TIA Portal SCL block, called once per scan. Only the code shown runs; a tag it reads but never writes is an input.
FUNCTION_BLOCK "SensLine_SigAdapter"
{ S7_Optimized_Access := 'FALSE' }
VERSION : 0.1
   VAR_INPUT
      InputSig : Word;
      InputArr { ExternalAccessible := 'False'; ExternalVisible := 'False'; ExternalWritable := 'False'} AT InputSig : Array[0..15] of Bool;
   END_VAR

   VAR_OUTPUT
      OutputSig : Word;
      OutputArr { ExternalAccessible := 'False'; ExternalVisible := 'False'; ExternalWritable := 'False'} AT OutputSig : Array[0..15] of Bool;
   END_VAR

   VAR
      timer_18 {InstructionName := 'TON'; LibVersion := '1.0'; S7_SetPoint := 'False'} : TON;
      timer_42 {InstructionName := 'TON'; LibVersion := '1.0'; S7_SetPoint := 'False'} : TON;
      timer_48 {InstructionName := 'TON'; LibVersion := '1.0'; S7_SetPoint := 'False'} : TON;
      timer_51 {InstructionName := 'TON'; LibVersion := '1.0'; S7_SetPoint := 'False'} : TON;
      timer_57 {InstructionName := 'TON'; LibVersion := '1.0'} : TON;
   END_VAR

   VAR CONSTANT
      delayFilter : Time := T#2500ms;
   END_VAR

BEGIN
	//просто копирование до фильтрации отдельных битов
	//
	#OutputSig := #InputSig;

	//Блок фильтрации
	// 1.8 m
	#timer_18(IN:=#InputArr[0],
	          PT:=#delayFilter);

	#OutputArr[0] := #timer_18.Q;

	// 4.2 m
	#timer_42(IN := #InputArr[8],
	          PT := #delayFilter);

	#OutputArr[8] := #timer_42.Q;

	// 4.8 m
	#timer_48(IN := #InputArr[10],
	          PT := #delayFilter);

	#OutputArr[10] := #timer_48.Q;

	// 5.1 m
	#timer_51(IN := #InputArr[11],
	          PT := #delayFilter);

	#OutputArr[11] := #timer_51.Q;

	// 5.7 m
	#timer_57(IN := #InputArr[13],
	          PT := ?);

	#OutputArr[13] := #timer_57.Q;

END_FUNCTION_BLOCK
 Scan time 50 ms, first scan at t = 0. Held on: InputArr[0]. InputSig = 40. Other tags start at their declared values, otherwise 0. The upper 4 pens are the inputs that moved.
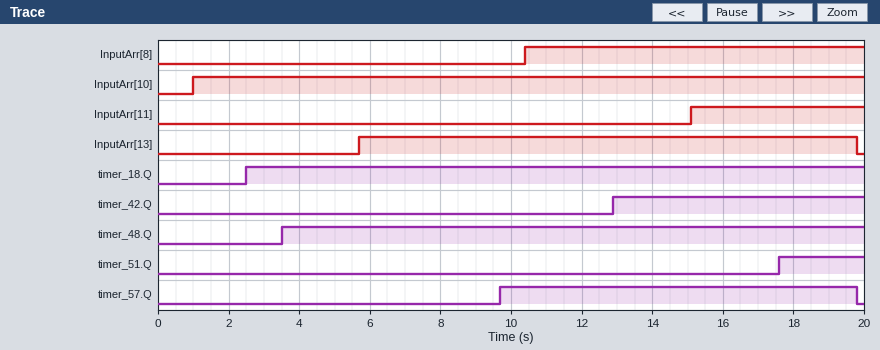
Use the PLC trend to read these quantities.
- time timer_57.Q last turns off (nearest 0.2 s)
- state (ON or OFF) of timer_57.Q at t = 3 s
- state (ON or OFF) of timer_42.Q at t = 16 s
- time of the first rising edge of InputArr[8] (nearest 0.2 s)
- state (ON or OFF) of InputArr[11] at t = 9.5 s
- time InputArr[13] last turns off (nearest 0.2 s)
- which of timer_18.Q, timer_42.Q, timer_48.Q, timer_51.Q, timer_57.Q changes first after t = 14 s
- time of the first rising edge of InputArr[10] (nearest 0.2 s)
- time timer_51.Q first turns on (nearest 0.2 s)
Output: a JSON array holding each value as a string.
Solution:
["19.8 s", "OFF", "ON", "10.4 s", "OFF", "19.8 s", "timer_51.Q", "1.0 s", "17.6 s"]
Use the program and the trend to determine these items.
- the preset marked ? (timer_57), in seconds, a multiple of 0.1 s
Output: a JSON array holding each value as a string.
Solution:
["4.0 s"]
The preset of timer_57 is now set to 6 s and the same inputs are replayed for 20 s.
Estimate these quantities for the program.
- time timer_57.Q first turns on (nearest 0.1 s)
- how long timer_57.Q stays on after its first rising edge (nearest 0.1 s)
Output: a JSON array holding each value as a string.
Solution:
["11.7 s", "8.1 s"]
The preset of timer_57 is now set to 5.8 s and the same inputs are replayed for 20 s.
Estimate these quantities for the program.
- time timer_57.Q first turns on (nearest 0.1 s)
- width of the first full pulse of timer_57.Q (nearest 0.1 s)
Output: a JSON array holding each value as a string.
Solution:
["11.5 s", "8.3 s"]
